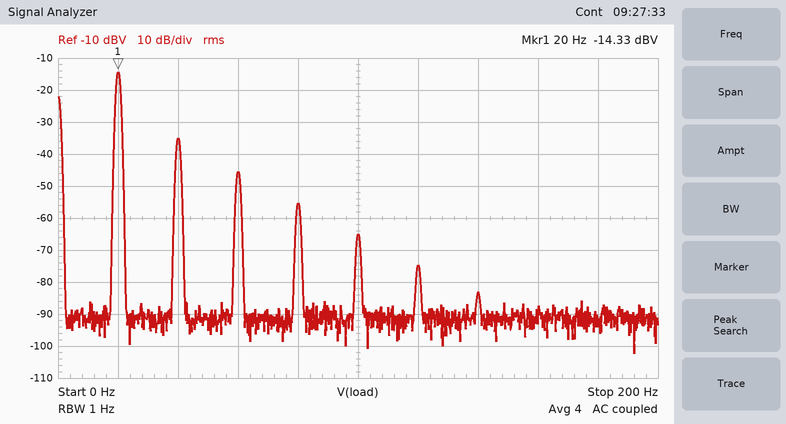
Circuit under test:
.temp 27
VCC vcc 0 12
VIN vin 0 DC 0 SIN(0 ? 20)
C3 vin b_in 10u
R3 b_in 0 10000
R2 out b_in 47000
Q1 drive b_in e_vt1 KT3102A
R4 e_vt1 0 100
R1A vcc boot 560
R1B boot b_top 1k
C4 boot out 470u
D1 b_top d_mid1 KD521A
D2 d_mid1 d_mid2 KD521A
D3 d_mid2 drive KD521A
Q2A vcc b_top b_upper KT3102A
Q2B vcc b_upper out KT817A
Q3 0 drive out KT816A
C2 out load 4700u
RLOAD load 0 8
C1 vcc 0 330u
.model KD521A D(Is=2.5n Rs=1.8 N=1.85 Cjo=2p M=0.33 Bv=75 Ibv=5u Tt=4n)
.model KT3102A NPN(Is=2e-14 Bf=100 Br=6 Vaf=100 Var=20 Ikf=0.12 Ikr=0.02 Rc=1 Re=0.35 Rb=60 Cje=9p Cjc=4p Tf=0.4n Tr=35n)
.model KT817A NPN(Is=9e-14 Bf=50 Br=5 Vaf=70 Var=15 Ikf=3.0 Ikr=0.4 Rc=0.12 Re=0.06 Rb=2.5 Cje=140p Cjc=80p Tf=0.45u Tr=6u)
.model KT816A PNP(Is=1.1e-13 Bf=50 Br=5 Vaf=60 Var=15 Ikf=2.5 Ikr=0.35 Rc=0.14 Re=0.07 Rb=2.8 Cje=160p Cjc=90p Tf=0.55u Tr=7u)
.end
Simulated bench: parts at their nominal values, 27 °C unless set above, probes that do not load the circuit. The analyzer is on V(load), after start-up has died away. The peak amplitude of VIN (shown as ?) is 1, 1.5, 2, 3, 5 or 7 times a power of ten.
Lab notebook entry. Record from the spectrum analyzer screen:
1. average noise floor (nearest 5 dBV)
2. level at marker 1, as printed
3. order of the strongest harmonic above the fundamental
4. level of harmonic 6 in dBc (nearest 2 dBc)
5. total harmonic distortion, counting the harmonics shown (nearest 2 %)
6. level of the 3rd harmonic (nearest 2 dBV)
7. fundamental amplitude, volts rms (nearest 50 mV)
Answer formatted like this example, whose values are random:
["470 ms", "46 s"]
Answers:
["-90 dBV", "-14.33 dBV", "2", "-60 dBc", "10 %", "-46 dBV", "200 mV"]
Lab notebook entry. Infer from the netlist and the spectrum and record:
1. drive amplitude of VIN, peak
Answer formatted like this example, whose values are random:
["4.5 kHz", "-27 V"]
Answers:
["50 mV"]
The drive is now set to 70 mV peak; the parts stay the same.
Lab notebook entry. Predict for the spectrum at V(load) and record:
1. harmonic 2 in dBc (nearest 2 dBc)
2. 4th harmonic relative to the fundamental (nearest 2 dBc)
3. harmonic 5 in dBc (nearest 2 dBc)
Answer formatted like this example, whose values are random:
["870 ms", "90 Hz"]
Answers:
["-16 dBc", "-30 dBc", "-36 dBc"]
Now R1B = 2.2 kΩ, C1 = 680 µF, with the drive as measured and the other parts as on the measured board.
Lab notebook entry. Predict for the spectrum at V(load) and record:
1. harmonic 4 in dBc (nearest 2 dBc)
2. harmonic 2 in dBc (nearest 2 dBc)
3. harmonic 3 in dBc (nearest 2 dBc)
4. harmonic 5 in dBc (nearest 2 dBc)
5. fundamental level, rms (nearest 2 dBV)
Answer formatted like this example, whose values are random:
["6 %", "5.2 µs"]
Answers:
["-22 dBc", "-12 dBc", "-16 dBc", "-26 dBc", "-14 dBV"]
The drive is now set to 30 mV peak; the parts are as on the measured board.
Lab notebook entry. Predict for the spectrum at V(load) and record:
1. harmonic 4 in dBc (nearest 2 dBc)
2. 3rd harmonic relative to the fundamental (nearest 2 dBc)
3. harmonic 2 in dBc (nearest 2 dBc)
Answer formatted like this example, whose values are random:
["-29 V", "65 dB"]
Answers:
["-56 dBc", "-42 dBc", "-26 dBc"]
